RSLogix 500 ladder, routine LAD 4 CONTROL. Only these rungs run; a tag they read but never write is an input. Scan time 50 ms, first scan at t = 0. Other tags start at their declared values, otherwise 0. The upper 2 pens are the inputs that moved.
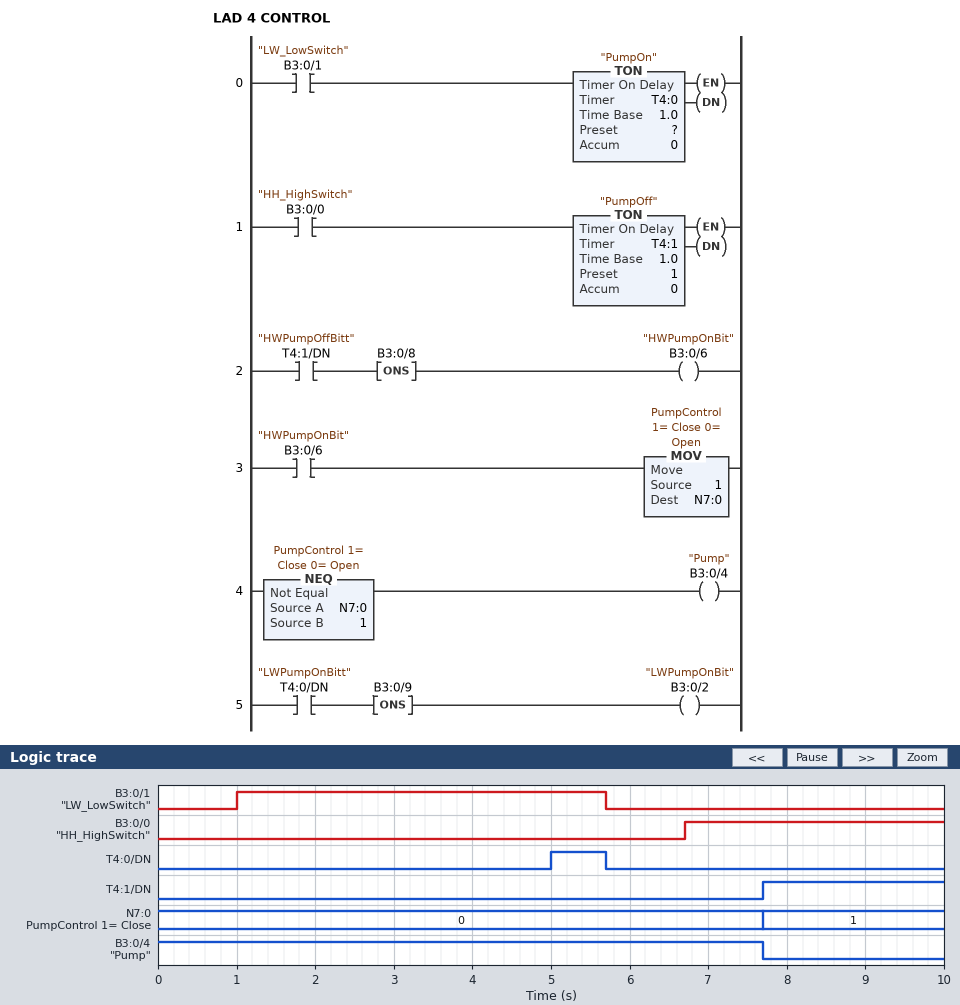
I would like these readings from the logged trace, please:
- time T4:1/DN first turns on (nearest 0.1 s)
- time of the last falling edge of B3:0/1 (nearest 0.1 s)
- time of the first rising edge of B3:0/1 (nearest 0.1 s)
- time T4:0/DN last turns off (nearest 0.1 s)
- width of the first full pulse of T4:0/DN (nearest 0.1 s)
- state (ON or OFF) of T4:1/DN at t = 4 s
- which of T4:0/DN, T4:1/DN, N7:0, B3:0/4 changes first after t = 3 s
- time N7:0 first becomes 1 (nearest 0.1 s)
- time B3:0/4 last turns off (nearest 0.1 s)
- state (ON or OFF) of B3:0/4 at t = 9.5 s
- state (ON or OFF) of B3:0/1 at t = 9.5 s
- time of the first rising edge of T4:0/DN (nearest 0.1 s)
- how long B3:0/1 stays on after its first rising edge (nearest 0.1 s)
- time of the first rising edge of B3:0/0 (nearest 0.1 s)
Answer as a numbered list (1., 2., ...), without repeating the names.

1. 7.7 s
2. 5.7 s
3. 1.0 s
4. 5.7 s
5. 0.7 s
6. OFF
7. T4:0/DN
8. 7.7 s
9. 7.7 s
10. OFF
11. OFF
12. 5.0 s
13. 4.7 s
14. 6.7 s
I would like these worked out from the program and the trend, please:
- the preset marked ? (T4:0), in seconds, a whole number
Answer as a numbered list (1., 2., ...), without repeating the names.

1. 4 s
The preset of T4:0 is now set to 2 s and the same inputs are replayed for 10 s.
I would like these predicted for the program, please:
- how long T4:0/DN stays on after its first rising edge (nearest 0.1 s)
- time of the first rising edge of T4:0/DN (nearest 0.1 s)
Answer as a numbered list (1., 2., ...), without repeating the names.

1. 2.7 s
2. 3.0 s
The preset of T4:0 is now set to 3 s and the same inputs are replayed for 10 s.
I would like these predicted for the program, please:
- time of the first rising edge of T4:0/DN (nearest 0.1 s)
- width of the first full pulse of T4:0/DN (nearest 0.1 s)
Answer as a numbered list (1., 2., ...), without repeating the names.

1. 4.0 s
2. 1.7 s
